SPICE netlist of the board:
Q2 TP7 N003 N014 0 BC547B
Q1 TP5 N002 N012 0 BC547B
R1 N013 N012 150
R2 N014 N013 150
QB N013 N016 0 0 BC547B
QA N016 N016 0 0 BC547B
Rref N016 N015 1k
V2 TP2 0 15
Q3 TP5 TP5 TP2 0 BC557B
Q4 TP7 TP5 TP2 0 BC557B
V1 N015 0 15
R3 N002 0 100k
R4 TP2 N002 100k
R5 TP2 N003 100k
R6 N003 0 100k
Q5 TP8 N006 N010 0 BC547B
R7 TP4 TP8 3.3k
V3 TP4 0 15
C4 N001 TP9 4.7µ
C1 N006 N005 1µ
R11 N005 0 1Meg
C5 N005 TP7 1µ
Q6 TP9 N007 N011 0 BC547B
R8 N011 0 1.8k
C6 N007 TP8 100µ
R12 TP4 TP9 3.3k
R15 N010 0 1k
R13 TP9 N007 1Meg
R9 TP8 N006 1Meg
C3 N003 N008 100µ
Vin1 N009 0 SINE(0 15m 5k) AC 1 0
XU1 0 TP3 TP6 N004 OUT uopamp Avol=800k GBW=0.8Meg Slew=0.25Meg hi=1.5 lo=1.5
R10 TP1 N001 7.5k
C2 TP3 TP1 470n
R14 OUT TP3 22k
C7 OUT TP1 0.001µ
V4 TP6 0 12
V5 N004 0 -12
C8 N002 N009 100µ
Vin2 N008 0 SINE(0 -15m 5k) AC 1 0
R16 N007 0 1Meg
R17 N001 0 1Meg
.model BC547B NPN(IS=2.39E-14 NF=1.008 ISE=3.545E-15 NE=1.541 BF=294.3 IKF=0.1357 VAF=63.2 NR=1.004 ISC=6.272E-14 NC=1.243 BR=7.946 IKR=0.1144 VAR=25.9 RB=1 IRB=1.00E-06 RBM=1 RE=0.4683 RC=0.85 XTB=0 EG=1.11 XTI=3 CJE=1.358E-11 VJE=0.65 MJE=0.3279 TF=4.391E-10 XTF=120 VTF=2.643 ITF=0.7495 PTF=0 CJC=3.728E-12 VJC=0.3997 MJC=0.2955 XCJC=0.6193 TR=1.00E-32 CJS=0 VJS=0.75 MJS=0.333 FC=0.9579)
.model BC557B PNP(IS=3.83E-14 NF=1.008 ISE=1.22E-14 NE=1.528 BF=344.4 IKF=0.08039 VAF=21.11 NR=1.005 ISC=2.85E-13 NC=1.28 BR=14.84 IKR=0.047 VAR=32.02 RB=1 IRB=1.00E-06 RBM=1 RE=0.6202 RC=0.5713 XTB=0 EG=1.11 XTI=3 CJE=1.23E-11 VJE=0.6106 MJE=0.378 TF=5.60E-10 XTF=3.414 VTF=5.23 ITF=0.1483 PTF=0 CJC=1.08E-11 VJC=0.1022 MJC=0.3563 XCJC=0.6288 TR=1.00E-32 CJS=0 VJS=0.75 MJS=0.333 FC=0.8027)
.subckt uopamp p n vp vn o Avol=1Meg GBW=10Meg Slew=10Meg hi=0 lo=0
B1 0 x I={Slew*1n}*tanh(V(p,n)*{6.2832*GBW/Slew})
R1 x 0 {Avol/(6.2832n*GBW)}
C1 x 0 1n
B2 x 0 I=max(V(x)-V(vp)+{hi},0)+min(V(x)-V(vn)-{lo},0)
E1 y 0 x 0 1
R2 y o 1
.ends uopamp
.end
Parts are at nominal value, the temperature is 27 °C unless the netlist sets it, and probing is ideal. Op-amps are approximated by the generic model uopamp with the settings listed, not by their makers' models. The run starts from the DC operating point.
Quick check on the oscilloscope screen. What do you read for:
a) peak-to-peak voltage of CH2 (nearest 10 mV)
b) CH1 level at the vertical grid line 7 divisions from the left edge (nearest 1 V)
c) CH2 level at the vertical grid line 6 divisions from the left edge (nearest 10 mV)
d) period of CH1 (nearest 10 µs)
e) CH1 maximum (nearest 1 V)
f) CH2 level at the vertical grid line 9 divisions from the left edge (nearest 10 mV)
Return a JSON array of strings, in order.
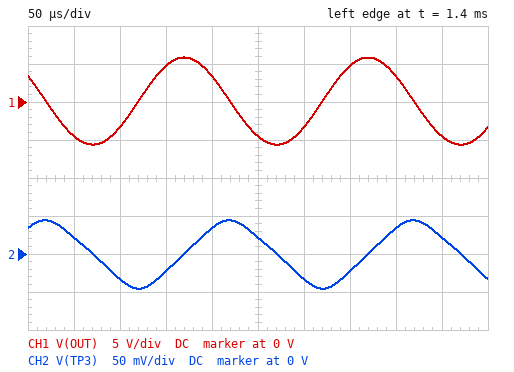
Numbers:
["90 mV", "5 V", "-30 mV", "200 µs", "6 V", "20 mV"]
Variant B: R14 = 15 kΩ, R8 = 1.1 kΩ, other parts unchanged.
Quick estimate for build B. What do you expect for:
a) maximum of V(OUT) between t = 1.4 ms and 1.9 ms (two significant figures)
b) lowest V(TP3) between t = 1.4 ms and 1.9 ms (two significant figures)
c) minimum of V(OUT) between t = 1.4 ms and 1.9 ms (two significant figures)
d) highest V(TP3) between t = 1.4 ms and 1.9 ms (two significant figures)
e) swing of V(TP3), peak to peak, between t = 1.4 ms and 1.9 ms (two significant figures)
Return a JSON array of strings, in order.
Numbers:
["7.1 V", "-68 mV", "-6.6 V", "66 mV", "130 mV"]
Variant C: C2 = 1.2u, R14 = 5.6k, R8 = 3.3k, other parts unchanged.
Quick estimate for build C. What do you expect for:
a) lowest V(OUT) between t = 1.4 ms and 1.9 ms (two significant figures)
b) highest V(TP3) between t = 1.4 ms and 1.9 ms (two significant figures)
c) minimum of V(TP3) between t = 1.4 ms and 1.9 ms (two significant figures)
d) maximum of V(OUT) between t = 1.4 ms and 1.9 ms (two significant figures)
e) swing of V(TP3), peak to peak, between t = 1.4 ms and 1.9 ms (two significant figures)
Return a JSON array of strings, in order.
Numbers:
["-940 mV", "6.1 mV", "-6.1 mV", "980 mV", "12 mV"]
